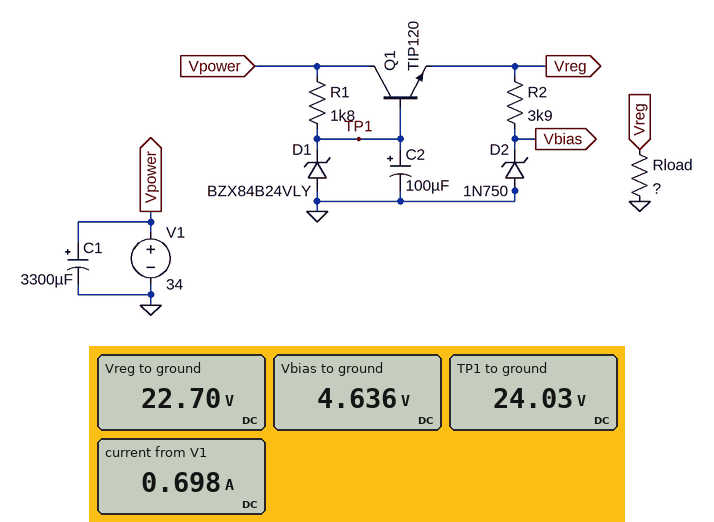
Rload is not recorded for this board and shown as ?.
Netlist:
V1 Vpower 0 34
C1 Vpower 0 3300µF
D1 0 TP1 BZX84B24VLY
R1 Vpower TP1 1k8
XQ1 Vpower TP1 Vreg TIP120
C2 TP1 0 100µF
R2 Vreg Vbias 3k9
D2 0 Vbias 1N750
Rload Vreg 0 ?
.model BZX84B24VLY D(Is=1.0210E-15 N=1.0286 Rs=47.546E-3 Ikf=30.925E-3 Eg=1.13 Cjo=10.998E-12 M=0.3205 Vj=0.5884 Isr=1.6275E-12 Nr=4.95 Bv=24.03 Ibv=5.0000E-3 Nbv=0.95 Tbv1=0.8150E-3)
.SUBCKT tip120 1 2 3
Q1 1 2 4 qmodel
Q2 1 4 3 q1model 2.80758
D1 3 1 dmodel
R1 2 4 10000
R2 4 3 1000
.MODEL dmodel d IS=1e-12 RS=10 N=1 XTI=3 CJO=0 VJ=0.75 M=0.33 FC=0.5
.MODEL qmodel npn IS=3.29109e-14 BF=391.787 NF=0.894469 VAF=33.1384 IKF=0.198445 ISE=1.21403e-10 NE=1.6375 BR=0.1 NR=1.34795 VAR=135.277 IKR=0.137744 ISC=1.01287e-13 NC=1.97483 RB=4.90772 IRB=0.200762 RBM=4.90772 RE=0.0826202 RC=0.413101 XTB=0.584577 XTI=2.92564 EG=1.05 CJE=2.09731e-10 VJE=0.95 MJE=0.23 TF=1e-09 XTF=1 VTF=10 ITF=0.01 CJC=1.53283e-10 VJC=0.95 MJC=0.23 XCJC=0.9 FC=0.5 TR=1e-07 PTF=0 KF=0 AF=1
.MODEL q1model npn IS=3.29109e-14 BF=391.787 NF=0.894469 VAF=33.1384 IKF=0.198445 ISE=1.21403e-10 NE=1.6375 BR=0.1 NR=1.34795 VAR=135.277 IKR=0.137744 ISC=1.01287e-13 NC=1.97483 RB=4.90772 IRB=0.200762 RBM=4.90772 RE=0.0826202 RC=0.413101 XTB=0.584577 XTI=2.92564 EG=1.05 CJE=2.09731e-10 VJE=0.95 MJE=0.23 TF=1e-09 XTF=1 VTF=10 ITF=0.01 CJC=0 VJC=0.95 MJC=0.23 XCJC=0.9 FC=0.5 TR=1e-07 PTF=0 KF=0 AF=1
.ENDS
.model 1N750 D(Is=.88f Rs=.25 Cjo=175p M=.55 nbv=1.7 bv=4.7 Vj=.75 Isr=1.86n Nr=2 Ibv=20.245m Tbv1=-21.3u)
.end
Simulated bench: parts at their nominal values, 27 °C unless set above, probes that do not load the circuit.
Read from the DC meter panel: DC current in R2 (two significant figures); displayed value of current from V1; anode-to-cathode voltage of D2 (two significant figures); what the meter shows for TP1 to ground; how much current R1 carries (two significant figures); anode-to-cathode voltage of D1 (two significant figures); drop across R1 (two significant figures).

4.6 mA
0.698 A
-4.6 V
24.03 V
5.5 mA
-24 V
10 V
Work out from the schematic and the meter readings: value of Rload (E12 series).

33 Ω
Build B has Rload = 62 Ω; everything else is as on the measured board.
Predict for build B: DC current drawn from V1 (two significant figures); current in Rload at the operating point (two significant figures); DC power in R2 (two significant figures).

380 mA
370 mA
84 mW
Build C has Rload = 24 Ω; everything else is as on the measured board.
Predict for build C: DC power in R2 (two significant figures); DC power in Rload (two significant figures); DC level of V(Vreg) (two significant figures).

83 mW
21 W
23 V
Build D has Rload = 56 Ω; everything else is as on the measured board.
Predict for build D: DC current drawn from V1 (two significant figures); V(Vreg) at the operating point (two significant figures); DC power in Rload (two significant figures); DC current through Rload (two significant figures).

420 mA
23 V
9.2 W
410 mA
